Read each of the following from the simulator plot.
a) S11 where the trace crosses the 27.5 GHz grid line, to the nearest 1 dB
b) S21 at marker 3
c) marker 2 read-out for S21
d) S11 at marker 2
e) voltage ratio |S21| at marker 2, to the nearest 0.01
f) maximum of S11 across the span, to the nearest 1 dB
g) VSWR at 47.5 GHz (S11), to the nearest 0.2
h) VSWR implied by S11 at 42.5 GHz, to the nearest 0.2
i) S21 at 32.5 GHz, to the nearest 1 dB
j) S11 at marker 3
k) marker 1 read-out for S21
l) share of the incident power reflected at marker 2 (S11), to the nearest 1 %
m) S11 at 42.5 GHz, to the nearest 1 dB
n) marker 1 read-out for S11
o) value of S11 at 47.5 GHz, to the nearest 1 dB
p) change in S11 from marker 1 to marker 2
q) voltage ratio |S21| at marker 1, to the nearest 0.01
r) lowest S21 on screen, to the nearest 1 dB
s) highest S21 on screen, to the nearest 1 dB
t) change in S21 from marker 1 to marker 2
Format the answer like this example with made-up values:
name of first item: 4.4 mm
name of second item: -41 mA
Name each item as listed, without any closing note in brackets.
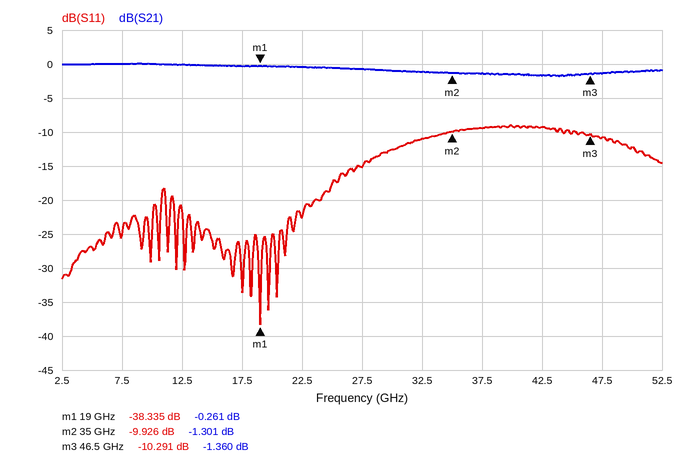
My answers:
S11 where the trace crosses the 27.5 GHz grid line, to the nearest 1 dB: -15 dB
S21 at marker 3: -1.360 dB
marker 2 read-out for S21: -1.301 dB
S11 at marker 2: -9.926 dB
voltage ratio |S21| at marker 2, to the nearest 0.01: 0.86
maximum of S11 across the span, to the nearest 1 dB: -9 dB
VSWR at 47.5 GHz (S11), to the nearest 0.2: 1.8
VSWR implied by S11 at 42.5 GHz, to the nearest 0.2: 2.0
S21 at 32.5 GHz, to the nearest 1 dB: -1 dB
S11 at marker 3: -10.291 dB
marker 1 read-out for S21: -0.261 dB
share of the incident power reflected at marker 2 (S11), to the nearest 1 %: 10 %
S11 at 42.5 GHz, to the nearest 1 dB: -9 dB
marker 1 read-out for S11: -38.335 dB
value of S11 at 47.5 GHz, to the nearest 1 dB: -11 dB
change in S11 from marker 1 to marker 2: 28.409 dB
voltage ratio |S21| at marker 1, to the nearest 0.01: 0.97
lowest S21 on screen, to the nearest 1 dB: -2 dB
highest S21 on screen, to the nearest 1 dB: 0 dB
change in S21 from marker 1 to marker 2: -1.040 dB
